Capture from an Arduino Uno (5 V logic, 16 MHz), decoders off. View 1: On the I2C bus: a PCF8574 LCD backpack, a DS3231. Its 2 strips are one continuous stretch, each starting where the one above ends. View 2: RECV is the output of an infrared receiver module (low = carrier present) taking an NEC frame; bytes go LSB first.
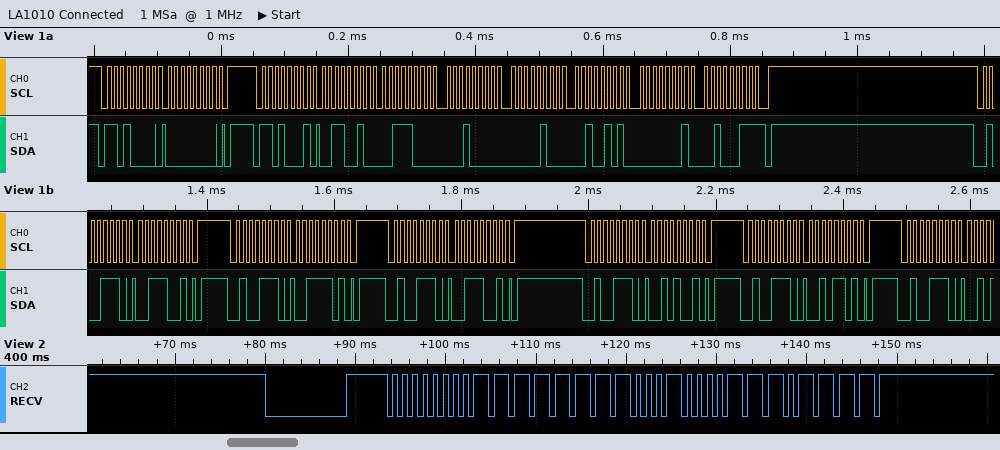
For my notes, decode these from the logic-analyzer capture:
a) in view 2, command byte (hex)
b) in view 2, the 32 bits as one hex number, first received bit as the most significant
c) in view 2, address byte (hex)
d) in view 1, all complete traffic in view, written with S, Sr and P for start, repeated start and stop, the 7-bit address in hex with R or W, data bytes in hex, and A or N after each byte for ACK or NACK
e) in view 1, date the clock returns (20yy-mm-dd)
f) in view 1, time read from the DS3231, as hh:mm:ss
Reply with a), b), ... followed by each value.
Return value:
a) 0x08
b) 0x00FF10EF
c) 0x00
d) S 68W A 00 A P S 68R A 32 A 38 A 10 A 04 A 25 A 01 A 23 N P S 27W A 39 A P S 27W A 3D A P S 27W A 39 A P S 27W A 29 A P S 27W A 2D A P S 27W A
e) 2023-01-25
f) 10:38:32
